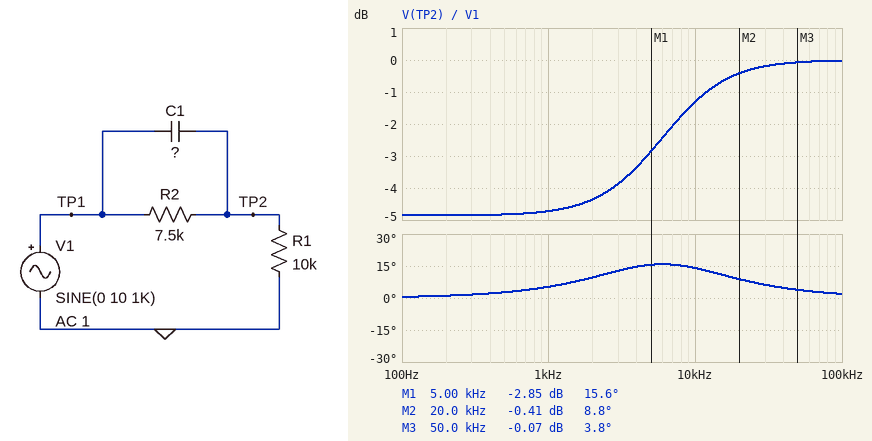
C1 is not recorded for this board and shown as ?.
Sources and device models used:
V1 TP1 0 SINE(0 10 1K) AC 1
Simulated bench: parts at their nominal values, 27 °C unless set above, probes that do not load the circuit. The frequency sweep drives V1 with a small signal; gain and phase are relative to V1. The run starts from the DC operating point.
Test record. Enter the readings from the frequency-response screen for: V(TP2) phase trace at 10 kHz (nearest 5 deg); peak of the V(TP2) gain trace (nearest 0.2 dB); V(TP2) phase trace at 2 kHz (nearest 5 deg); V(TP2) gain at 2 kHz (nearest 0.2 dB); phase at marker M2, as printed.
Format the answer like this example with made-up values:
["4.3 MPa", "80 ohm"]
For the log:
["15 deg", "0 dB", "10 deg", "-4.4 dB", "8.8 deg"]
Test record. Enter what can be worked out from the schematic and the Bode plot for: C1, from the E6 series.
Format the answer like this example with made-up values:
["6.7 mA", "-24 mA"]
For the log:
["4.7 nF"]
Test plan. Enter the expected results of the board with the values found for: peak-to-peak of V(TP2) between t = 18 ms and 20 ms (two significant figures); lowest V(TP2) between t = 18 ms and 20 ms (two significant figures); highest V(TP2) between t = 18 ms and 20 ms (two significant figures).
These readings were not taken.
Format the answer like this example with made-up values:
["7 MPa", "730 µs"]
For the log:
["12 V", "-5.8 V", "5.8 V"]
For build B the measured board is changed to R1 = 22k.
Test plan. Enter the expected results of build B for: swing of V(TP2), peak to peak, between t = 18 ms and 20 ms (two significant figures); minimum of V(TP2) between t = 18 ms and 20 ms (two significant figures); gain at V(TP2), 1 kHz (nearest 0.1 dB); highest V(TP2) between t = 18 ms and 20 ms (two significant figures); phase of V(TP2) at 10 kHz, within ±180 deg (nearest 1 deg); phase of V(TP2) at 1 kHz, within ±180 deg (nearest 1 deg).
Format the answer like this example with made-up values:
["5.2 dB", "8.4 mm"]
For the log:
["15 V", "-7.5 V", "-2.5 dB", "7.5 V", "7 deg", "3 deg"]
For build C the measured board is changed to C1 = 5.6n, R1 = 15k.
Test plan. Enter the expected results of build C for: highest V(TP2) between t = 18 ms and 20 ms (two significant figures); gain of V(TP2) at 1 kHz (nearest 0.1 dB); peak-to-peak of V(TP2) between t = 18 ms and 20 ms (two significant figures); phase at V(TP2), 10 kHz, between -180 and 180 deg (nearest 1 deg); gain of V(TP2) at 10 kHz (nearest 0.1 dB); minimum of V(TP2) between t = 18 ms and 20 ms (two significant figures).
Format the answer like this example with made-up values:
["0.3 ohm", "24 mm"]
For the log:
["6.8 V", "-3.4 dB", "14 V", "9 deg", "-0.6 dB", "-6.8 V"]
